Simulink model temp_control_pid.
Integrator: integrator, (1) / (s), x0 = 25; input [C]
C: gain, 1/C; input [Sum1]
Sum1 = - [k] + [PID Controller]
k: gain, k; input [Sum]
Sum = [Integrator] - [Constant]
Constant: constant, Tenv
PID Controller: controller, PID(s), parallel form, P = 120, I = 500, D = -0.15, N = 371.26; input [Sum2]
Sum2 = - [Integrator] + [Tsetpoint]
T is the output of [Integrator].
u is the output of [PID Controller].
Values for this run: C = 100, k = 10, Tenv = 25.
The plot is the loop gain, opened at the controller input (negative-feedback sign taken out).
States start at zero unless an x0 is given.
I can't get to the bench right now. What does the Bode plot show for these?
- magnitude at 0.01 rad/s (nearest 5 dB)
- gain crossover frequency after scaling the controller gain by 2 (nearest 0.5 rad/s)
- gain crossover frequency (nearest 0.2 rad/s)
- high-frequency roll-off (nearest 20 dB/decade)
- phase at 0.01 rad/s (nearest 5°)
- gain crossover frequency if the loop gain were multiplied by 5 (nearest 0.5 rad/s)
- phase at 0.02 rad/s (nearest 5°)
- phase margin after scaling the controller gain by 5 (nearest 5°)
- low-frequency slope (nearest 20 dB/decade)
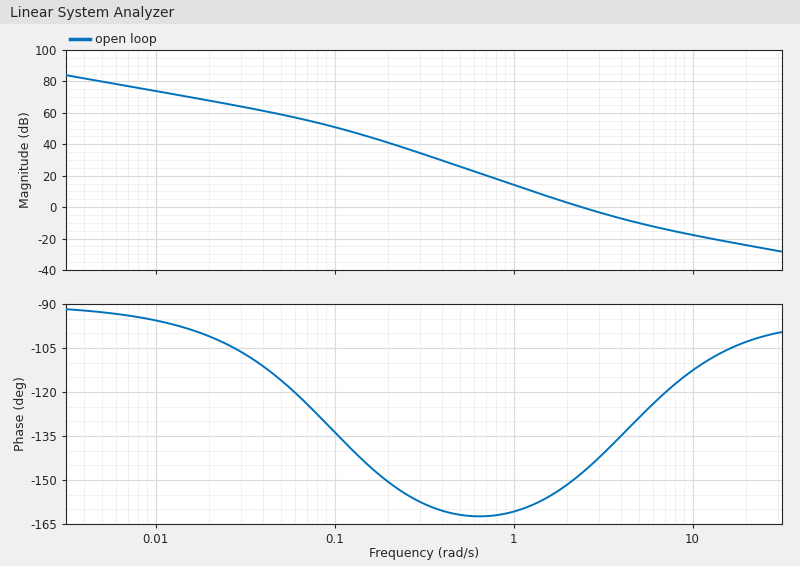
75 dB
3.5 rad/s
2.4 rad/s
-20 dB/decade
-95°
7.0 rad/s
-100°
60°
-20 dB/decade
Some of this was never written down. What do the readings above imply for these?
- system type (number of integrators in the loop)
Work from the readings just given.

1
